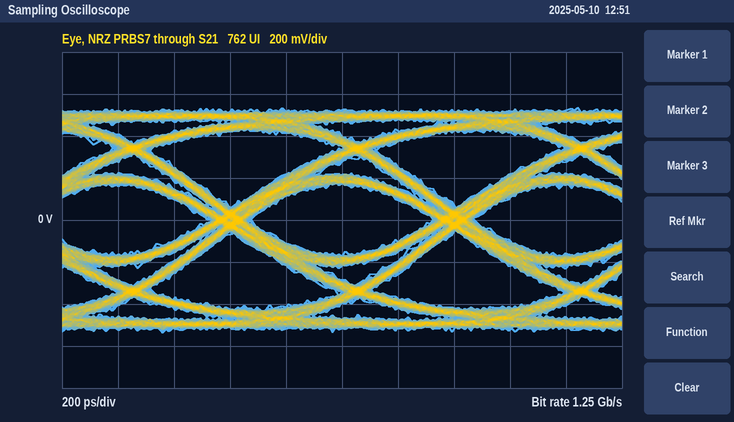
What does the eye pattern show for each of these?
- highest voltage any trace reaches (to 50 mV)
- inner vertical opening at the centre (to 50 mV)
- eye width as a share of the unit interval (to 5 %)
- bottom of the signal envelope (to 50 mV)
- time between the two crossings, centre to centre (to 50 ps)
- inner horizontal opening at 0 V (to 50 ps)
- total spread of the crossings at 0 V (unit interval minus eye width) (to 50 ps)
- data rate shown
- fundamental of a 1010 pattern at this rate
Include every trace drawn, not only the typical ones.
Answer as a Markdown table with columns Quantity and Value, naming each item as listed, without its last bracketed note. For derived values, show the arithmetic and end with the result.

| Quantity | Value |
|---|---|
| highest voltage any trace reaches | 550 mV |
| inner vertical opening at the centre | 350 mV |
| eye width as a share of the unit interval | 650 ps / 800 ps ≈ 81.2 %, so 80 % to the nearest 5 % |
| bottom of the signal envelope | -550 mV |
| time between the two crossings, centre to centre | 800 ps |
| inner horizontal opening at 0 V | 650 ps |
| total spread of the crossings at 0 V (unit interval minus eye width) | 150 ps |
| data rate shown | 1.25 Gb/s |
| fundamental of a 1010 pattern at this rate | 625 MHz |
